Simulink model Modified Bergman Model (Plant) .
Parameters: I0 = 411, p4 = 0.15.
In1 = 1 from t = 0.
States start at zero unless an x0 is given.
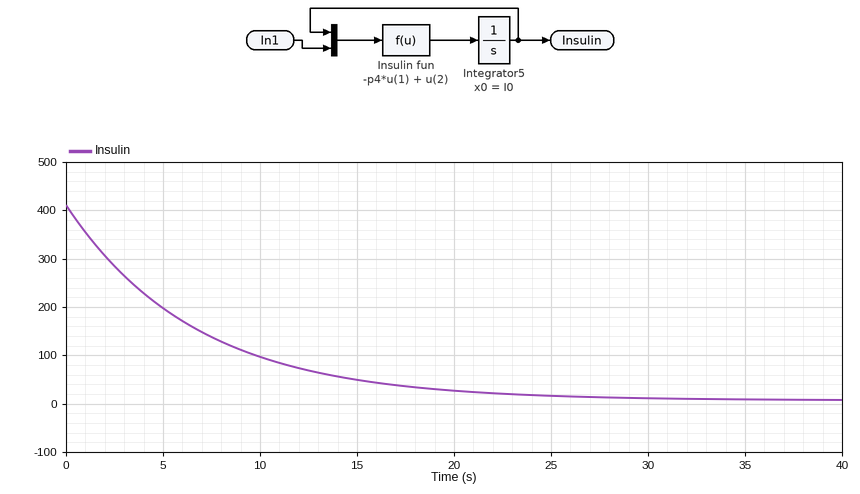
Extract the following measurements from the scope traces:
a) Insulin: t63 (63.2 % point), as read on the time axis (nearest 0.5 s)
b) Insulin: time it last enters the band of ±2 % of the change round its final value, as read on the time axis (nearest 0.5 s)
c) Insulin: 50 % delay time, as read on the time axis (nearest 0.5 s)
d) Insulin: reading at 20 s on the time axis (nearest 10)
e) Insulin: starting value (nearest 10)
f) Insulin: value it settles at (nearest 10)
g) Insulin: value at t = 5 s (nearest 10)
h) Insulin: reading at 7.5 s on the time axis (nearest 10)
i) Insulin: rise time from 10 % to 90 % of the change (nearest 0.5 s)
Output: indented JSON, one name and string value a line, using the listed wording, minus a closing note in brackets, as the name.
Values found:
{
  "Insulin: t63 (63.2 % point), as read on the time axis": "6.5 s",
  "Insulin: time it last enters the band of ±2 % of the change round its final value, as read on the time axis": "26.0 s",
  "Insulin: 50 % delay time, as read on the time axis": "4.5 s",
  "Insulin: reading at 20 s on the time axis": "30",
  "Insulin: starting value": "410",
  "Insulin: value it settles at": "10",
  "Insulin: value at t = 5 s": "200",
  "Insulin: reading at 7.5 s on the time axis": "140",
  "Insulin: rise time from 10 % to 90 % of the change": "14.5 s"
}
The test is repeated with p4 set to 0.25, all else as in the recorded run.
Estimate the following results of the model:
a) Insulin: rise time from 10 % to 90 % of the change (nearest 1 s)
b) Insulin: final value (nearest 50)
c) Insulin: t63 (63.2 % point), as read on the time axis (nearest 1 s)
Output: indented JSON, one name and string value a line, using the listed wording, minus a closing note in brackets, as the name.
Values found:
{
  "Insulin: rise time from 10 % to 90 % of the change": "9 s",
  "Insulin: final value": "0",
  "Insulin: t63 (63.2 % point), as read on the time axis": "4 s"
}
